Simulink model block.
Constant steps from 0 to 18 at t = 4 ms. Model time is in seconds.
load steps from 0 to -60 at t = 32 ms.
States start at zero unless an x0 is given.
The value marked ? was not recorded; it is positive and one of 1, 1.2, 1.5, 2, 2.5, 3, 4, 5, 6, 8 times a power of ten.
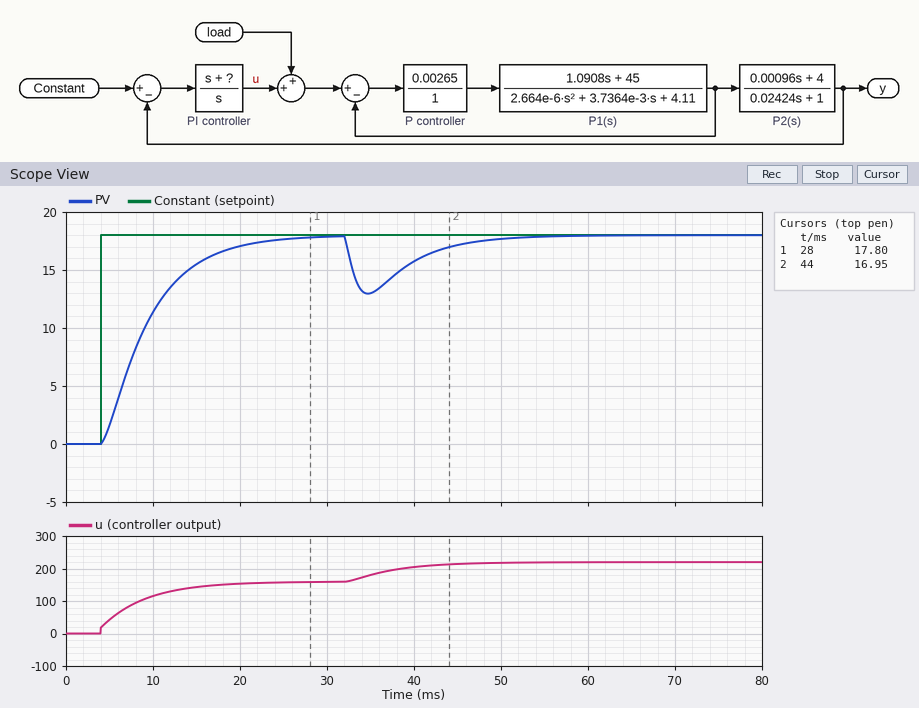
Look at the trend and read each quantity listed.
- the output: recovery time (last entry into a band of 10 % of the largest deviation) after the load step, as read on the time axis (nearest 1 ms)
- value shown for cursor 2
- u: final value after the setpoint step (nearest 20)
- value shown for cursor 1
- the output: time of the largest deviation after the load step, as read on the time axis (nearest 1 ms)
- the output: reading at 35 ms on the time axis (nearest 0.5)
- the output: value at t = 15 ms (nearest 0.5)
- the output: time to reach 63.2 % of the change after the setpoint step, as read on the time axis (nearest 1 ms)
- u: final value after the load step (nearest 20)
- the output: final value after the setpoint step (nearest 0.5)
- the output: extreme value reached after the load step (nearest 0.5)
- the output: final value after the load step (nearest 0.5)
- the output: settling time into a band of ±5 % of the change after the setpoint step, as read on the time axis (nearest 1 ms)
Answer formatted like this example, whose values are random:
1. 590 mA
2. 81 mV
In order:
1. 48 ms
2. 16.95
3. 160
4. 17.80
5. 35 ms
6. 13.0
7. 15.5
8. 10 ms
9. 220
10. 18.0
11. 13.0
12. 18.0
13. 20 ms
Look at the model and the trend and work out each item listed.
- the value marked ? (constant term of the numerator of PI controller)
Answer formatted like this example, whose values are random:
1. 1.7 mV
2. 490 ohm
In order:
1. 1500
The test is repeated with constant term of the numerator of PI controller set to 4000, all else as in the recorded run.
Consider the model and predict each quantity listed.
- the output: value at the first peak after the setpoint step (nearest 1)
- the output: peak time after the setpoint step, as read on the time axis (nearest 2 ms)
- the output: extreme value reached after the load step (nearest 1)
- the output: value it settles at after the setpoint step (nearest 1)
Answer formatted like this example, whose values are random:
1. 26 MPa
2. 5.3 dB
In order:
1. 19
2. 10 ms
3. 14
4. 18
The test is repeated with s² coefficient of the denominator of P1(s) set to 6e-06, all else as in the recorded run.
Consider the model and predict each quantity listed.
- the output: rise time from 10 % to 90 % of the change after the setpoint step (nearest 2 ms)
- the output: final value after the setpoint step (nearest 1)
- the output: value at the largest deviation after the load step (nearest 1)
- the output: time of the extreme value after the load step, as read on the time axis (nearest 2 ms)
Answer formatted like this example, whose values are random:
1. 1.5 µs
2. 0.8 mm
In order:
1. 12 ms
2. 18
3. 12
4. 36 ms
